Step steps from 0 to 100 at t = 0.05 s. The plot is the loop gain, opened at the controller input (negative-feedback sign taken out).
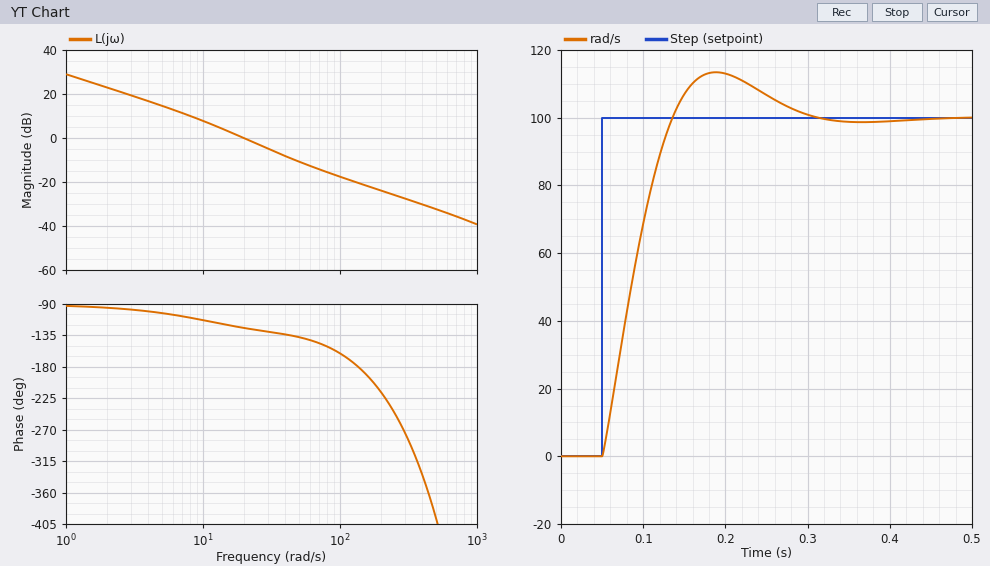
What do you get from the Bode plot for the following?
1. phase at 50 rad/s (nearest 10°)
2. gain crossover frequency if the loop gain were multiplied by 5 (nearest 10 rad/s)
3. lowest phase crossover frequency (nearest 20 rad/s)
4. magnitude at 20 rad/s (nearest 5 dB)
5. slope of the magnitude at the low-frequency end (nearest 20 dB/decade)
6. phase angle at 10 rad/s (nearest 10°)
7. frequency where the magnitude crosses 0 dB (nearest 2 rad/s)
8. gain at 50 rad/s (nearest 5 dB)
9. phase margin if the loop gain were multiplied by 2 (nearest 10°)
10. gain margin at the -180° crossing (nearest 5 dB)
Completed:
-140°
70 rad/s
140 rad/s
0 dB
-20 dB/decade
-110°
20 rad/s
-10 dB
50°
20 dB
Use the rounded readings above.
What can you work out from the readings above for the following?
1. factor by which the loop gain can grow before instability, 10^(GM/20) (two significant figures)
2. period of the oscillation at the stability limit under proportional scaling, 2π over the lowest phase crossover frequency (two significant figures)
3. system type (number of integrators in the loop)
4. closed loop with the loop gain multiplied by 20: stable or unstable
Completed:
10
0.045 s
1
unstable
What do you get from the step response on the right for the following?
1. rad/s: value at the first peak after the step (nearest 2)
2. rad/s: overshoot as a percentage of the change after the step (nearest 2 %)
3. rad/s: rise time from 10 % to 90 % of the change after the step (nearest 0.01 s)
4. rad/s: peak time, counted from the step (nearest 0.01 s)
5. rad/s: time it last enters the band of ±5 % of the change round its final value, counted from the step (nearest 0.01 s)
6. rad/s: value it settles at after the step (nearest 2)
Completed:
114
14 %
0.06 s
0.14 s
0.21 s
100
